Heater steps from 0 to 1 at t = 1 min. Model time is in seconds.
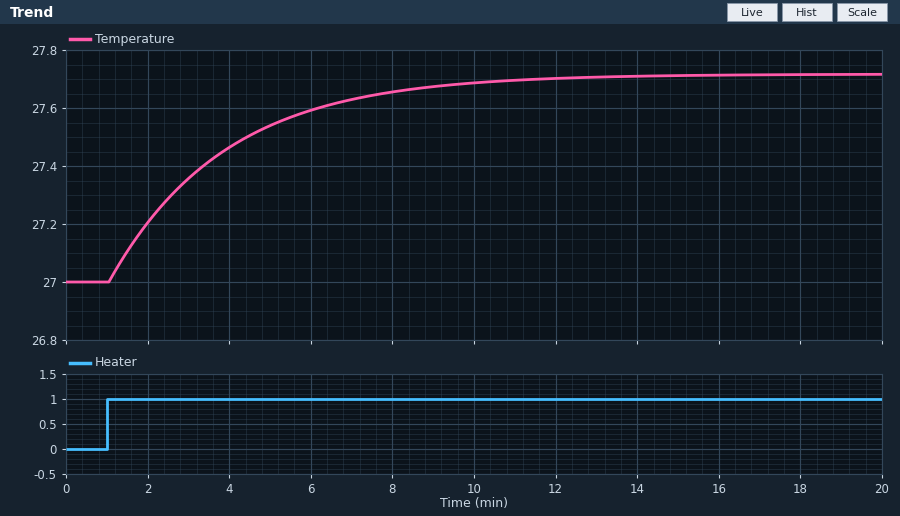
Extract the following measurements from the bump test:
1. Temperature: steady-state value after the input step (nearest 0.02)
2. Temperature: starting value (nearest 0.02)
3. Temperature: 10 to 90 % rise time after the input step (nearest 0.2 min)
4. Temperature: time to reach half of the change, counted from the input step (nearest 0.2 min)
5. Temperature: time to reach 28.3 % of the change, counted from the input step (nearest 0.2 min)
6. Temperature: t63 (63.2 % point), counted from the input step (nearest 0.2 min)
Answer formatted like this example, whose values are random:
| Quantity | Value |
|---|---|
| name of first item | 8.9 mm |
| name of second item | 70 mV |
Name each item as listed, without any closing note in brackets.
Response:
| Quantity | Value |
|---|---|
| Temperature: steady-state value after the input step | 27.72 |
| Temperature: starting value | 27.00 |
| Temperature: 10 to 90 % rise time after the input step | 6.2 min |
| Temperature: time to reach half of the change, counted from the input step | 2.0 min |
| Temperature: time to reach 28.3 % of the change, counted from the input step | 1.0 min |
| Temperature: t63 (63.2 % point), counted from the input step | 2.8 min |
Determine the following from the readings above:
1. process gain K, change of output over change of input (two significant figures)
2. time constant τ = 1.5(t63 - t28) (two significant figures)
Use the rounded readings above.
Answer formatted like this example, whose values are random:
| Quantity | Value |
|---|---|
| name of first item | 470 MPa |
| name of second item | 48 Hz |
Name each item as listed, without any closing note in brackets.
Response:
| Quantity | Value |
|---|---|
| process gain K, change of output over change of input | 0.72 |
| time constant τ = 1.5(t63 - t28) | 2.7 min |
